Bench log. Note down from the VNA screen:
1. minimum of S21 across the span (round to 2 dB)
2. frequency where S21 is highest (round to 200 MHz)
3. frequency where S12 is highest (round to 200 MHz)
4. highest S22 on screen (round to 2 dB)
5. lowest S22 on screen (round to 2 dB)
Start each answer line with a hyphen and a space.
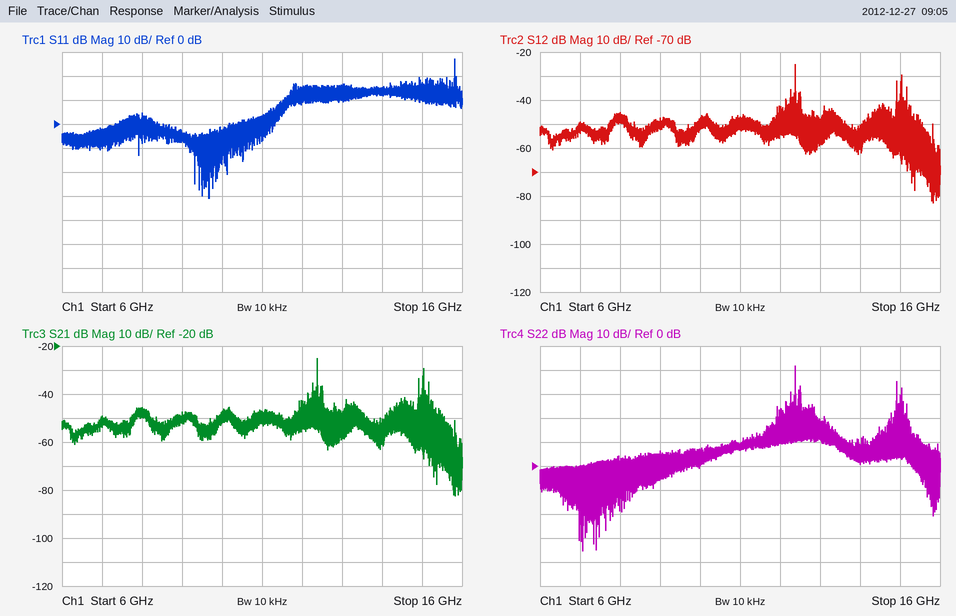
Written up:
- -82 dB
- 12.4 GHz
- 12.4 GHz
- 42 dB
- -36 dB
